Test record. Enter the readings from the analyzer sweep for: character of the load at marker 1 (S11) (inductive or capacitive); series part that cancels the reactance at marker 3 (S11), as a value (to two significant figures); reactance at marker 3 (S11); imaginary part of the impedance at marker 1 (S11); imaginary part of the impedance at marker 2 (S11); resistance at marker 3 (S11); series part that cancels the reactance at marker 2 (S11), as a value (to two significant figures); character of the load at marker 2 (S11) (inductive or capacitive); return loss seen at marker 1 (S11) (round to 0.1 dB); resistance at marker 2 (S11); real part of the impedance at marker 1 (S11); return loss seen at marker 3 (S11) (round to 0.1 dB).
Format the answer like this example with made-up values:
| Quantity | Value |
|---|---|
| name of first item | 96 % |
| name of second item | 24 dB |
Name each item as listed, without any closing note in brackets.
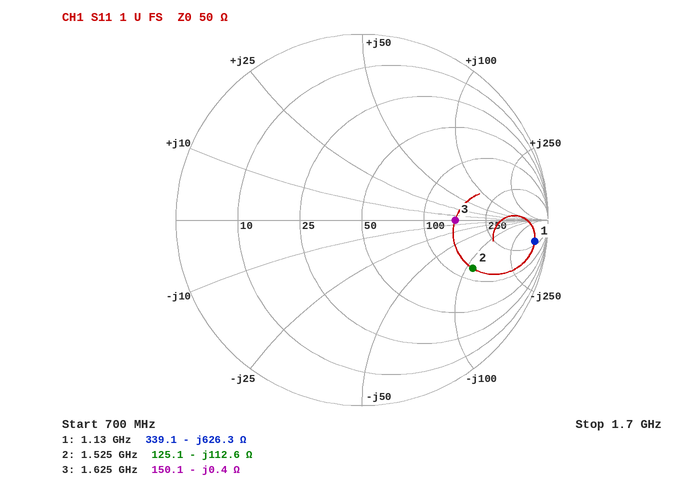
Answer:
| Quantity | Value |
|---|---|
| character of the load at marker 1 (S11) | capacitive |
| series part that cancels the reactance at marker 3 (S11), as a value | 39 pH |
| reactance at marker 3 | -0.4 Ω |
| imaginary part of the impedance at marker 1 | -626.3 Ω |
| imaginary part of the impedance at marker 2 | -112.6 Ω |
| resistance at marker 3 | 150.1 Ω |
| series part that cancels the reactance at marker 2 (S11), as a value | 12 nH |
| character of the load at marker 2 (S11) | capacitive |
| return loss seen at marker 1 (S11) | 0.6 dB |
| resistance at marker 2 | 125.1 Ω |
| real part of the impedance at marker 1 | 339.1 Ω |
| return loss seen at marker 3 (S11) | 6.0 dB |
